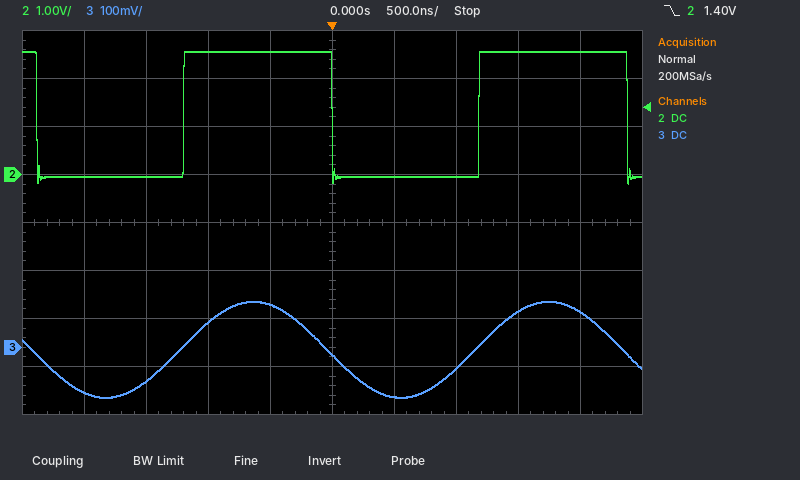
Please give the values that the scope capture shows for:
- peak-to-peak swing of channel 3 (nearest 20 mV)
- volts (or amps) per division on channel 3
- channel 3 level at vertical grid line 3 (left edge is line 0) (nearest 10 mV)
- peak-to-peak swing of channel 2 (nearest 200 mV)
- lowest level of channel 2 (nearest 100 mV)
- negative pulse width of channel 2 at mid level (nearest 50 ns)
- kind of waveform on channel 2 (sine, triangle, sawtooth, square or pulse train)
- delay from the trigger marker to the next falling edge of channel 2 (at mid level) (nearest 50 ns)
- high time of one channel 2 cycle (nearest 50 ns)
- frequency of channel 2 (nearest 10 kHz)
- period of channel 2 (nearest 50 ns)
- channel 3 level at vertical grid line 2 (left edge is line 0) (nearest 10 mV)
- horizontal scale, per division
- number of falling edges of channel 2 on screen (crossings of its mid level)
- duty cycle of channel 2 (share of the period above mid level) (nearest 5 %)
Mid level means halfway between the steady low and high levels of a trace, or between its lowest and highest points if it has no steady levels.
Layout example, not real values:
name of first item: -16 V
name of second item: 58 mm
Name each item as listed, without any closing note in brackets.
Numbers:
peak-to-peak swing of channel 3: 200 mV
volts (or amps) per division on channel 3: 100 mV
channel 3 level at vertical grid line 3 (left edge is line 0): 50 mV
peak-to-peak swing of channel 2: 2.8 V
lowest level of channel 2: -200 mV
negative pulse width of channel 2 at mid level: 1.20 µs
kind of waveform on channel 2: square
delay from the trigger marker to the next falling edge of channel 2 (at mid level): 2.40 µs
high time of one channel 2 cycle: 1.20 µs
frequency of channel 2: 420 kHz
period of channel 2: 2.40 µs
channel 3 level at vertical grid line 2 (left edge is line 0): -70 mV
horizontal scale, per division: 500 ns
number of falling edges of channel 2 on screen: 3
duty cycle of channel 2 (share of the period above mid level): 50 %
